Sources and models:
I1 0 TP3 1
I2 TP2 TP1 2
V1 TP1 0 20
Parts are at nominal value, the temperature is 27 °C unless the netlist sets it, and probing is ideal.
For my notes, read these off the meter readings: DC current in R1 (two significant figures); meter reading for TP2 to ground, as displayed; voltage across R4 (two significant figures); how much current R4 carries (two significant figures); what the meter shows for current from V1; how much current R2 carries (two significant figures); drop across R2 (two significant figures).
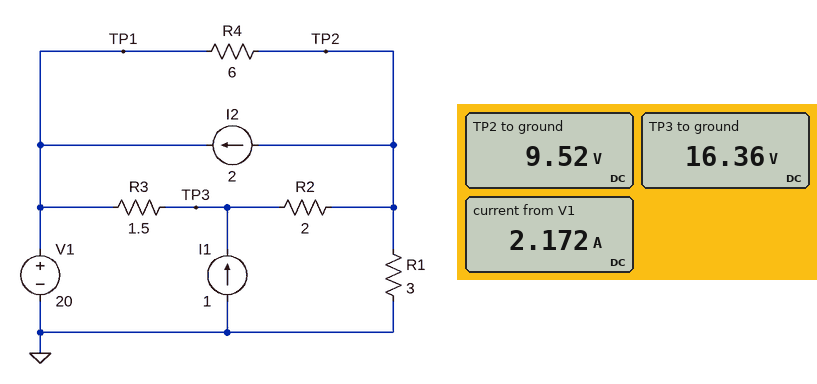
3.2 A
9.52 V
10 V
1.7 A
2.172 A
3.4 A
6.8 V
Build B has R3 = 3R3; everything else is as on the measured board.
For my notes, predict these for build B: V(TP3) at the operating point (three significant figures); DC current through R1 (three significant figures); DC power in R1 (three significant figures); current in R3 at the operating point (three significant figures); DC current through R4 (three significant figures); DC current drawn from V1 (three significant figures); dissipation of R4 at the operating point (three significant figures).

14.0 V
2.77 A
23.1 W
1.83 A
1.95 A
1.77 A
22.7 W
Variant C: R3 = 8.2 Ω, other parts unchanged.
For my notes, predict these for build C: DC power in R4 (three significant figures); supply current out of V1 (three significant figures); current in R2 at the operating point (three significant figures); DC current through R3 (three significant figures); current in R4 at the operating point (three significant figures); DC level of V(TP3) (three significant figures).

28.8 W
1.28 A
2.09 A
1.09 A
2.19 A
11.0 V
